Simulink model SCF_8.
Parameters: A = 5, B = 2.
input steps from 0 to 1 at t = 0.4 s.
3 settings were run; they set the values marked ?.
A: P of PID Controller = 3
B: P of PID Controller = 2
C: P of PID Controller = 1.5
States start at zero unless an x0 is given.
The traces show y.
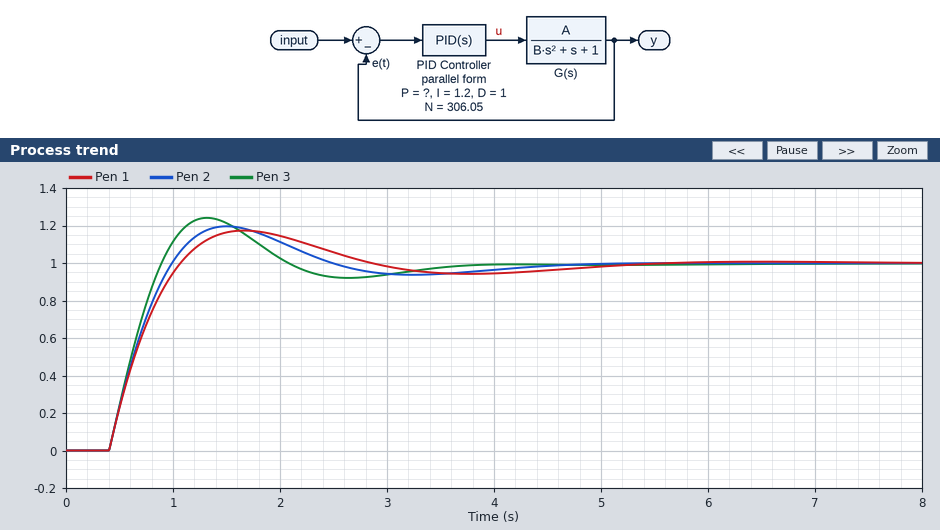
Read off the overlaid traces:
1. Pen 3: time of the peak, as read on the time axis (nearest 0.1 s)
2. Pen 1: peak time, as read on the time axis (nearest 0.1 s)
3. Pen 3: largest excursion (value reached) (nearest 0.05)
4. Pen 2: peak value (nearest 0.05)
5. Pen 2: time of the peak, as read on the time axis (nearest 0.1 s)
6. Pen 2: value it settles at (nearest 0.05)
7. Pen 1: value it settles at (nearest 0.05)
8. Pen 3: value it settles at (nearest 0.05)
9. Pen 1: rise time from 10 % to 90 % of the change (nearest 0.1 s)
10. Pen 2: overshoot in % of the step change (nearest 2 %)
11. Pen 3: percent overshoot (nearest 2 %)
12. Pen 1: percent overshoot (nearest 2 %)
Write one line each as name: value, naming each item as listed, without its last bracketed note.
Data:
Pen 3: time of the peak, as read on the time axis: 1.3 s
Pen 1: peak time, as read on the time axis: 1.7 s
Pen 3: largest excursion (value reached): 1.25
Pen 2: peak value: 1.20
Pen 2: time of the peak, as read on the time axis: 1.5 s
Pen 2: value it settles at: 1.00
Pen 1: value it settles at: 1.00
Pen 3: value it settles at: 1.00
Pen 1: rise time from 10 % to 90 % of the change: 0.5 s
Pen 2: overshoot in % of the step change: 20 %
Pen 3: percent overshoot: 24 %
Pen 1: percent overshoot: 18 %
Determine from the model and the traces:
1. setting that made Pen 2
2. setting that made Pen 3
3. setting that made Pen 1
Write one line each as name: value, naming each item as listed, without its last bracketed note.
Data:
setting that made Pen 2: B
setting that made Pen 3: A
setting that made Pen 1: C
